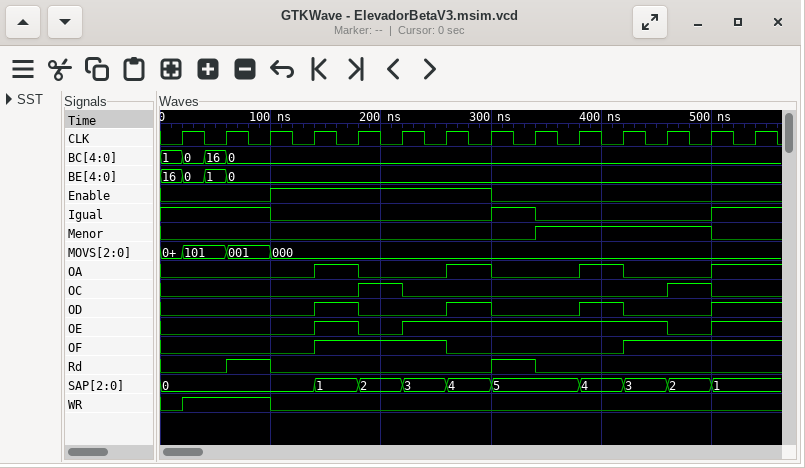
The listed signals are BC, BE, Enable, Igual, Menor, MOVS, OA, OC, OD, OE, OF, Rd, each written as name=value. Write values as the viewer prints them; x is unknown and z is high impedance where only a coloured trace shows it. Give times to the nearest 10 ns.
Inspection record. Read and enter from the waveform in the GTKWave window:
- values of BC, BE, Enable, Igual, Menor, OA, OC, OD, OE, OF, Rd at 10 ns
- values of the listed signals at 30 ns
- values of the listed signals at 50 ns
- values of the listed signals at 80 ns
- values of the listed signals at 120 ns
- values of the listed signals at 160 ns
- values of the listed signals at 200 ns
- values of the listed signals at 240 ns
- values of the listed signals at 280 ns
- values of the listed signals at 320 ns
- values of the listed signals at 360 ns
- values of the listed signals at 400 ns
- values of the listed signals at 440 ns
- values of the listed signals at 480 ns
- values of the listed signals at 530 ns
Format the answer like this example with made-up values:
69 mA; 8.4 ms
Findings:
BC=1, BE=16, Enable=0, Igual=1, Menor=0, OA=0, OC=0, OD=0, OE=0, OF=0, Rd=0; BC=0, BE=0, Enable=0, Igual=1, Menor=0, MOVS=101, OA=0, OC=0, OD=0, OE=0, OF=0, Rd=0; BC=16, BE=1, Enable=0, Igual=1, Menor=0, MOVS=101, OA=0, OC=0, OD=0, OE=0, OF=0, Rd=0; BC=0, BE=0, Enable=0, Igual=1, Menor=0, MOVS=001, OA=0, OC=0, OD=0, OE=0, OF=0, Rd=1; BC=0, BE=0, Enable=1, Igual=0, Menor=0, MOVS=000, OA=0, OC=0, OD=0, OE=0, OF=0, Rd=0; BC=0, BE=0, Enable=1, Igual=0, Menor=0, MOVS=000, OA=1, OC=0, OD=1, OE=1, OF=1, Rd=0; BC=0, BE=0, Enable=1, Igual=0, Menor=0, MOVS=000, OA=0, OC=1, OD=0, OE=0, OF=1, Rd=0; BC=0, BE=0, Enable=1, Igual=0, Menor=0, MOVS=000, OA=0, OC=0, OD=0, OE=1, OF=1, Rd=0; BC=0, BE=0, Enable=1, Igual=0, Menor=0, MOVS=000, OA=1, OC=0, OD=1, OE=1, OF=0, Rd=0; BC=0, BE=0, Enable=0, Igual=1, Menor=0, MOVS=000, OA=0, OC=0, OD=0, OE=1, OF=0, Rd=1; BC=0, BE=0, Enable=0, Igual=0, Menor=1, MOVS=000, OA=0, OC=0, OD=0, OE=1, OF=0, Rd=0; BC=0, BE=0, Enable=0, Igual=0, Menor=1, MOVS=000, OA=1, OC=0, OD=1, OE=1, OF=0, Rd=0; BC=0, BE=0, Enable=0, Igual=0, Menor=1, MOVS=000, OA=0, OC=0, OD=0, OE=1, OF=1, Rd=0; BC=0, BE=0, Enable=0, Igual=0, Menor=1, MOVS=000, OA=0, OC=1, OD=0, OE=0, OF=1, Rd=0; BC=0, BE=0, Enable=0, Igual=1, Menor=0, MOVS=000, OA=1, OC=0, OD=1, OE=1, OF=1, Rd=0
